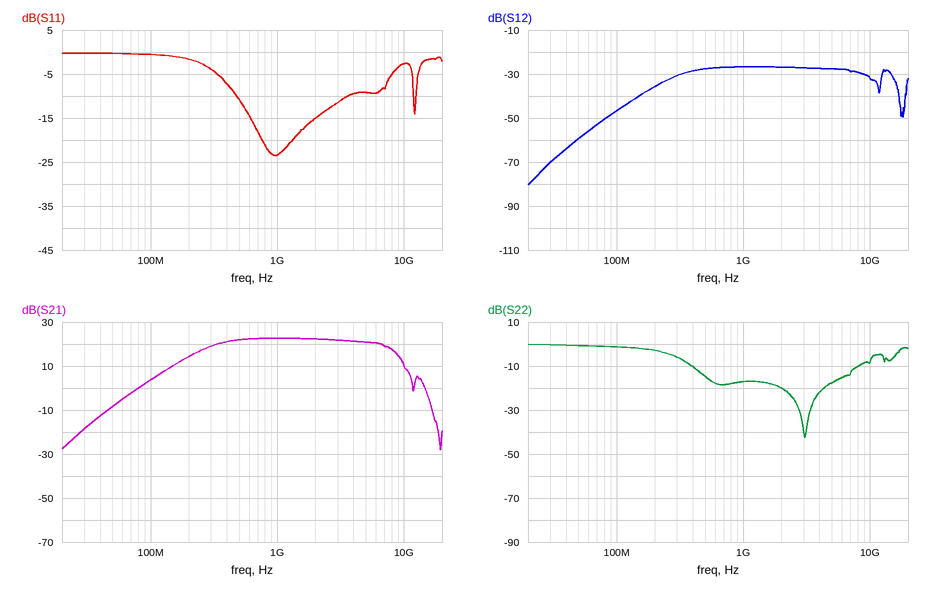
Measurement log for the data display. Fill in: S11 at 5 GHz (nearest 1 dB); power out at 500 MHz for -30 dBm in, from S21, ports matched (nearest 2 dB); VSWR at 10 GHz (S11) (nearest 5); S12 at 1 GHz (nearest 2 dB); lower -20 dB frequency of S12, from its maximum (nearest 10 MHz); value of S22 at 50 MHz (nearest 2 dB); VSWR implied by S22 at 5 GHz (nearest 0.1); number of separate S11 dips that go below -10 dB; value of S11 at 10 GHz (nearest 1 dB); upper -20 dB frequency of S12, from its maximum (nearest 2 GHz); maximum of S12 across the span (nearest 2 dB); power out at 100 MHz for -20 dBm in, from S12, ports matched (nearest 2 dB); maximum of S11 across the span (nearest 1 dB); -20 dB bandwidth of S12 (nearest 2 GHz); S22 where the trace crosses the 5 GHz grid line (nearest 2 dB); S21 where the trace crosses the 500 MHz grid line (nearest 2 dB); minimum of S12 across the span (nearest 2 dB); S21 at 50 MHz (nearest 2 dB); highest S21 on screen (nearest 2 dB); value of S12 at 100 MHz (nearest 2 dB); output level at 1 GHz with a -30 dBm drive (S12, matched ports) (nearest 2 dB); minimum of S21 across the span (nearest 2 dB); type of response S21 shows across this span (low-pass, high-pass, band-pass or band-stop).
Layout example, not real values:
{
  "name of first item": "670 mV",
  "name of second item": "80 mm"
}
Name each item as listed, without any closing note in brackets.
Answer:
{
  "S11 at 5 GHz": "-9 dB",
  "power out at 500 MHz for -30 dBm in, from S21, ports matched": "-8 dBm",
  "VSWR at 10 GHz (S11)": "5",
  "S12 at 1 GHz": "-26 dB",
  "lower -20 dB frequency of S12, from its maximum": "100 MHz",
  "value of S22 at 50 MHz": "0 dB",
  "VSWR implied by S22 at 5 GHz": "1.3",
  "number of separate S11 dips that go below -10 dB": "2",
  "value of S11 at 10 GHz": "-3 dB",
  "upper -20 dB frequency of S12, from its maximum": "18 GHz",
  "maximum of S12 across the span": "-26 dB",
  "power out at 100 MHz for -20 dBm in, from S12, ports matched": "-66 dBm",
  "maximum of S11 across the span": "0 dB",
  "-20 dB bandwidth of S12": "18 GHz",
  "S22 where the trace crosses the 5 GHz grid line": "-18 dB",
  "S21 where the trace crosses the 500 MHz grid line": "22 dB",
  "minimum of S12 across the span": "-80 dB",
  "S21 at 50 MHz": "-8 dB",
  "highest S21 on screen": "22 dB",
  "value of S12 at 100 MHz": "-46 dB",
  "output level at 1 GHz with a -30 dBm drive (S12, matched ports)": "-56 dBm",
  "minimum of S21 across the span": "-28 dB",
  "type of response S21 shows across this span": "band-pass"
}
